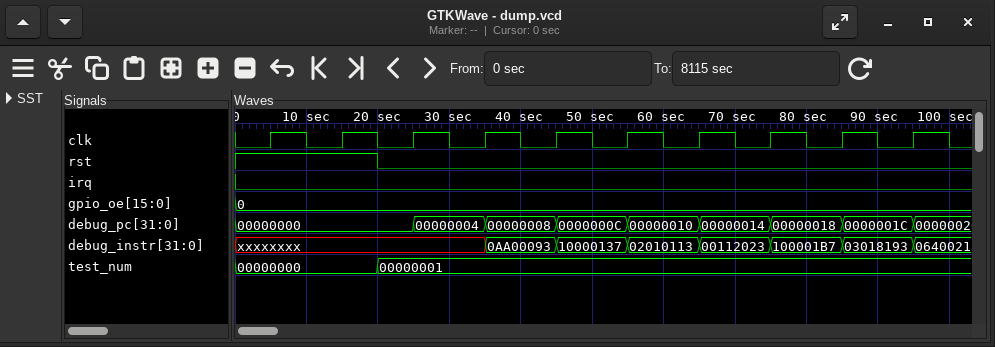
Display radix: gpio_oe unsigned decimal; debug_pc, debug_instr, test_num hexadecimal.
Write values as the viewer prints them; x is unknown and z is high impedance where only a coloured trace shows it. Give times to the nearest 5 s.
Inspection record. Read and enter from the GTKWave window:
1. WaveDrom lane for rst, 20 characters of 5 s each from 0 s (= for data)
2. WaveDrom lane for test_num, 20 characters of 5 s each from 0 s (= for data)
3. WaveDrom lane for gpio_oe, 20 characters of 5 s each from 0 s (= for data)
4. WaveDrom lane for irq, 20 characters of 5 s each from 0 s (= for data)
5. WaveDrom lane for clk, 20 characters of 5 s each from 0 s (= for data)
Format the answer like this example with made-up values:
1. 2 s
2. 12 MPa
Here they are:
1. {name: 'rst', wave: '1...0...............'}
2. {name: 'test_num', wave: '=...=...............', data: '00000000 00000001'}
3. {name: 'gpio_oe', wave: '=...................', data: '0'}
4. {name: 'irq', wave: '0...................'}
5. {name: 'clk', wave: '01010101010101010101'}
